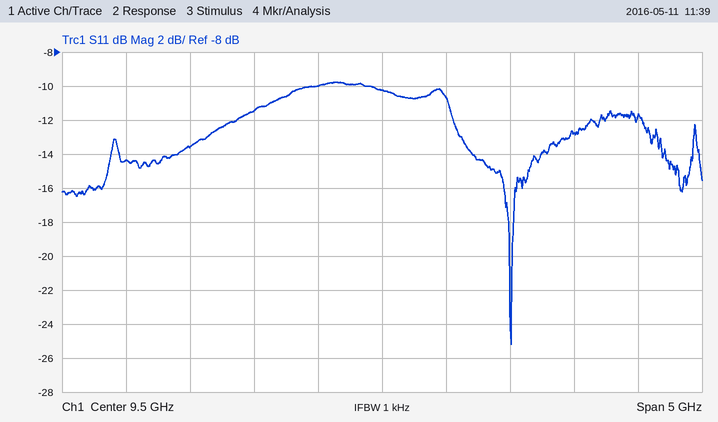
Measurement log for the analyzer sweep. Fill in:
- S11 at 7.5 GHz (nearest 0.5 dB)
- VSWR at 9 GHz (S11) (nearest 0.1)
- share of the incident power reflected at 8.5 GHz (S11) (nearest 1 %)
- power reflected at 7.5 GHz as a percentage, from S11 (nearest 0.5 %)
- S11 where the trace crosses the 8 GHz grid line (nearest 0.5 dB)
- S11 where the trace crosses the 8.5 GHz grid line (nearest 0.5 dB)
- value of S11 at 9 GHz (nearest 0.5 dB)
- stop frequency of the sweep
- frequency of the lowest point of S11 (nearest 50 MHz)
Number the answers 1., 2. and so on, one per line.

1. -14.5 dB
2. 1.9
3. 7 %
4. 3.5 %
5. -13.5 dB
6. -11.5 dB
7. -10.0 dB
8. 12 GHz
9. 10.50 GHz
